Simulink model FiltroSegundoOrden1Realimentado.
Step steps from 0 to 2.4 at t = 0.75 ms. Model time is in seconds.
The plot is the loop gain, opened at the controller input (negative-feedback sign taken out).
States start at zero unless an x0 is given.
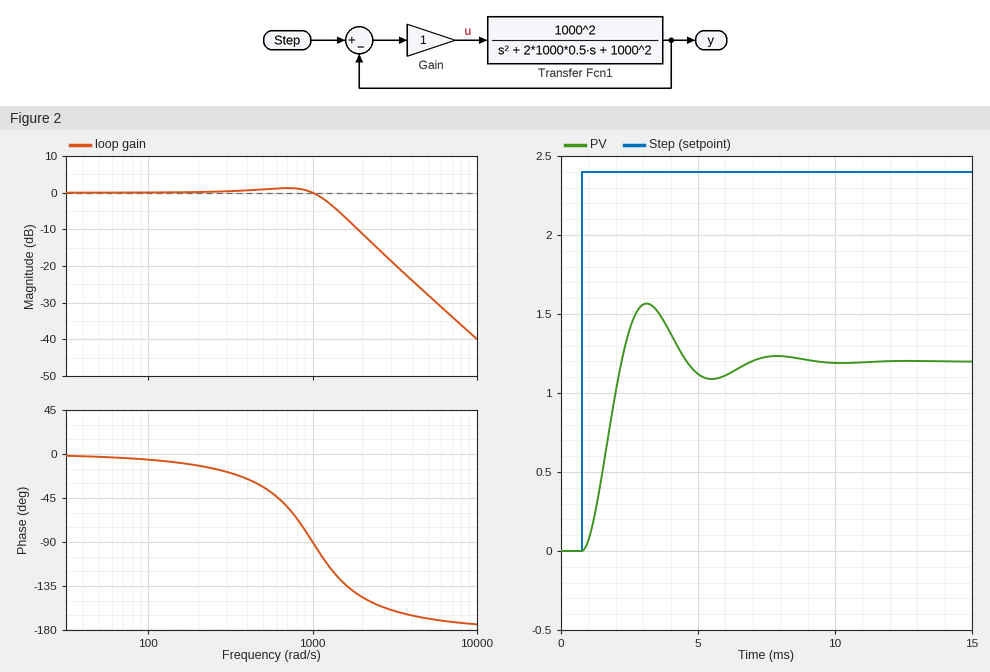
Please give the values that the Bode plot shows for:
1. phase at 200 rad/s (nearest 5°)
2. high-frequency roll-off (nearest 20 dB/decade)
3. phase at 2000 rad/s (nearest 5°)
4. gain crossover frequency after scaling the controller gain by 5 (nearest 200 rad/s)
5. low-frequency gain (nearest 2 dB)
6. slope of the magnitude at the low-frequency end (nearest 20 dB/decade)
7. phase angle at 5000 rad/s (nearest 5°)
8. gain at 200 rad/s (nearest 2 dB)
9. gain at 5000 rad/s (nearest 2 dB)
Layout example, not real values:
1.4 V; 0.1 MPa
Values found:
-10°; -40 dB/decade; -145°; 2400 rad/s; 0 dB; 0 dB/decade; -170°; 0 dB; -28 dB
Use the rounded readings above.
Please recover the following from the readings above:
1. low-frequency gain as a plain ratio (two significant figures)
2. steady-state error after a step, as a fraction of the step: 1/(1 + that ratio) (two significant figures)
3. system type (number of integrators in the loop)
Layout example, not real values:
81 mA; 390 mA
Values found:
1.0; 0.50; 0
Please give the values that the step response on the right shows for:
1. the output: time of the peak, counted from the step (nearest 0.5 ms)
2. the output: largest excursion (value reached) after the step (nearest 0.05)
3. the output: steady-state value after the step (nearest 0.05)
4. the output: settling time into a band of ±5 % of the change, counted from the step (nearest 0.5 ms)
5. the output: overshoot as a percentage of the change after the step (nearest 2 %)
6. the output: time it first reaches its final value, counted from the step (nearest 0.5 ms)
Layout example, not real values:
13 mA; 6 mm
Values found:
2.5 ms; 1.55; 1.20; 5.5 ms; 30 %; 1.5 ms
